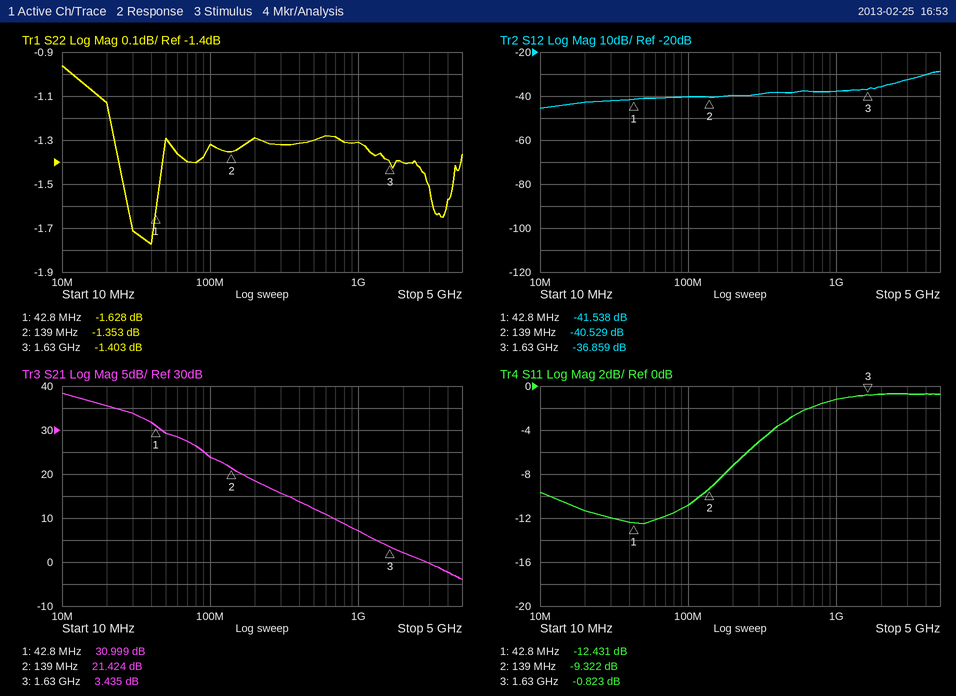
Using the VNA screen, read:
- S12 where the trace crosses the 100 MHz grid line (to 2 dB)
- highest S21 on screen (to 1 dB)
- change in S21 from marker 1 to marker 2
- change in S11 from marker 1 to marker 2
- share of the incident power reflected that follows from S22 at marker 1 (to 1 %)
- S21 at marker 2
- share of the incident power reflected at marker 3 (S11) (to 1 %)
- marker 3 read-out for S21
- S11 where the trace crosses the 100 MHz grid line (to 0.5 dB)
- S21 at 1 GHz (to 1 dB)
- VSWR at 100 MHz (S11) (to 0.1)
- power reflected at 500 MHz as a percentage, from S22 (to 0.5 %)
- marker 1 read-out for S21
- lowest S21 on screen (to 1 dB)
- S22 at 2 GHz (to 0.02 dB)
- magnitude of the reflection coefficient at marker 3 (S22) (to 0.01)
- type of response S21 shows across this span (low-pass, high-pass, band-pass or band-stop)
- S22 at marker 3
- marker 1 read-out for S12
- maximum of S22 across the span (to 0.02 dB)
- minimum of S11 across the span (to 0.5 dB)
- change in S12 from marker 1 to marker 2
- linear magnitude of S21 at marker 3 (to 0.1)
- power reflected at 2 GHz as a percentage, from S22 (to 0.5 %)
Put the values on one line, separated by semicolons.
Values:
-40 dB; 38 dB; -9.575 dB; 3.109 dB; 69 %; 21.424 dB; 83 %; 3.435 dB; -11.0 dB; 7 dB; 1.8; 74.0 %; 30.999 dB; -4 dB; -1.40 dB; 0.85; low-pass; -1.403 dB; -41.538 dB; -0.96 dB; -12.5 dB; 1.009 dB; 1.5; 72.5 %
